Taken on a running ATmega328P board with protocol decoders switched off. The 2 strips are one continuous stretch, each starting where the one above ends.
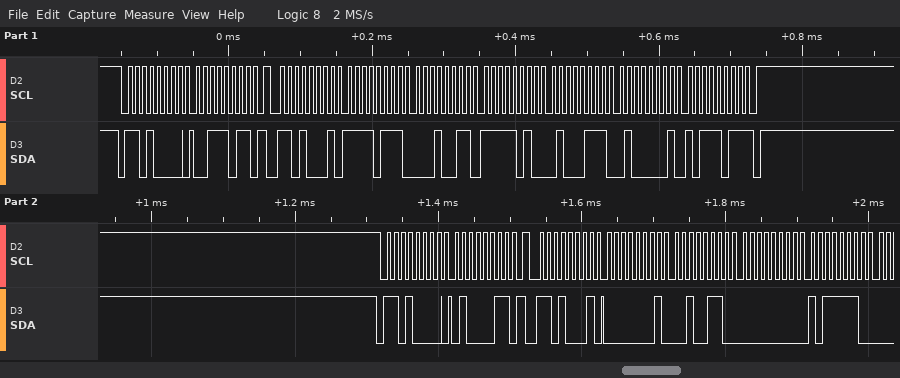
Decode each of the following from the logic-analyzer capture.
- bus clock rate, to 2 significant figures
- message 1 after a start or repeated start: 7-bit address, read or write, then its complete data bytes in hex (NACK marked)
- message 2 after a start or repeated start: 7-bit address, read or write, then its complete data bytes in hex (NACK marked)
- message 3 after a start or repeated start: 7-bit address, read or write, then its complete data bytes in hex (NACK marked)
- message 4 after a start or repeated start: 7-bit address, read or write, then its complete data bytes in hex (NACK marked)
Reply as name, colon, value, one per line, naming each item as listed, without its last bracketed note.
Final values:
bus clock rate, to 2 significant figures: 100 kHz
message 1 after a start or repeated start: 7-bit address, read or write, then its complete data bytes in hex: 0x68 write: 3B
message 2 after a start or repeated start: 7-bit address, read or write, then its complete data bytes in hex: 0x68 read: F7 13 FA 47 41 BB NACK
message 3 after a start or repeated start: 7-bit address, read or write, then its complete data bytes in hex: 0x68 write: 43
message 4 after a start or repeated start: 7-bit address, read or write, then its complete data bytes in hex: 0x68 read: 01 26 00 BE
